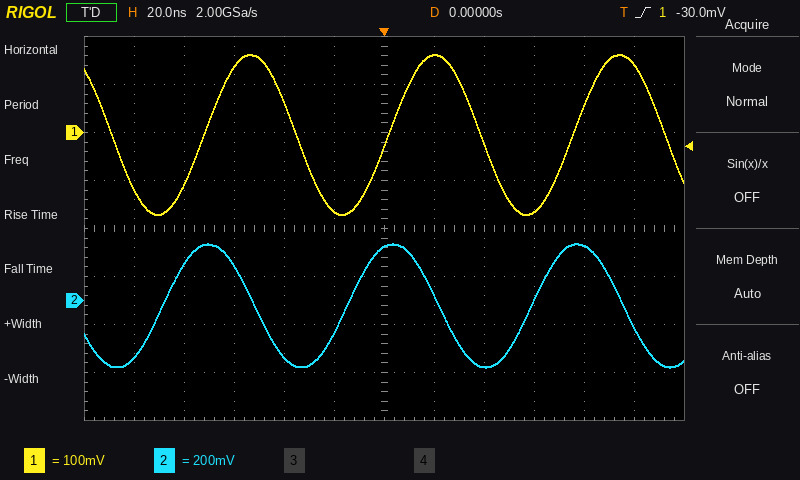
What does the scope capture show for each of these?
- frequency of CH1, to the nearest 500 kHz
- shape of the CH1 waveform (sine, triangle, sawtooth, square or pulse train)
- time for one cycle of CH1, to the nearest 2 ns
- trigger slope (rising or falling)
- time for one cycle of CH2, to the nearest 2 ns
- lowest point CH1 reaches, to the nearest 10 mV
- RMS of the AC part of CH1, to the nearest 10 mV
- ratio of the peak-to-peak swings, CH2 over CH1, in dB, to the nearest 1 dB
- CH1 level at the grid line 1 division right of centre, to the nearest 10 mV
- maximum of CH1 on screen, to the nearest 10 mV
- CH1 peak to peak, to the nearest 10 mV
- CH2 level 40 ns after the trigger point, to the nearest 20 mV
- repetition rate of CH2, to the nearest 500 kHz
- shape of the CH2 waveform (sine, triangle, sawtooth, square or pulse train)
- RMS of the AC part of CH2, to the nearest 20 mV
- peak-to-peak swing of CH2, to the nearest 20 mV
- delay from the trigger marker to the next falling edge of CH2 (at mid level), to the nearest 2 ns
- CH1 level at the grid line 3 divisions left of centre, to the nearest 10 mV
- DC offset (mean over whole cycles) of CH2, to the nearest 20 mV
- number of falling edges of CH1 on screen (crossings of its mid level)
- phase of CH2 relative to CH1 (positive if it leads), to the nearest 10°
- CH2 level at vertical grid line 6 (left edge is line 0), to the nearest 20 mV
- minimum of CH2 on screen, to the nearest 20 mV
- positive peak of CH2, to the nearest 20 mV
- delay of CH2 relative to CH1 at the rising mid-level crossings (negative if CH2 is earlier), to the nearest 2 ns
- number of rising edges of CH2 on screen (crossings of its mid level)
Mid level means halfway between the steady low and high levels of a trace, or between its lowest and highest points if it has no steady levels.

13.5 MHz
sine
74 ns
rising
74 ns
-170 mV
120 mV
4 dB
160 mV
160 mV
330 mV
-280 mV
13.5 MHz
sine
180 mV
520 mV
22 ns
140 mV
-20 mV
4
+80°
220 mV
-280 mV
240 mV
-16 ns
3
